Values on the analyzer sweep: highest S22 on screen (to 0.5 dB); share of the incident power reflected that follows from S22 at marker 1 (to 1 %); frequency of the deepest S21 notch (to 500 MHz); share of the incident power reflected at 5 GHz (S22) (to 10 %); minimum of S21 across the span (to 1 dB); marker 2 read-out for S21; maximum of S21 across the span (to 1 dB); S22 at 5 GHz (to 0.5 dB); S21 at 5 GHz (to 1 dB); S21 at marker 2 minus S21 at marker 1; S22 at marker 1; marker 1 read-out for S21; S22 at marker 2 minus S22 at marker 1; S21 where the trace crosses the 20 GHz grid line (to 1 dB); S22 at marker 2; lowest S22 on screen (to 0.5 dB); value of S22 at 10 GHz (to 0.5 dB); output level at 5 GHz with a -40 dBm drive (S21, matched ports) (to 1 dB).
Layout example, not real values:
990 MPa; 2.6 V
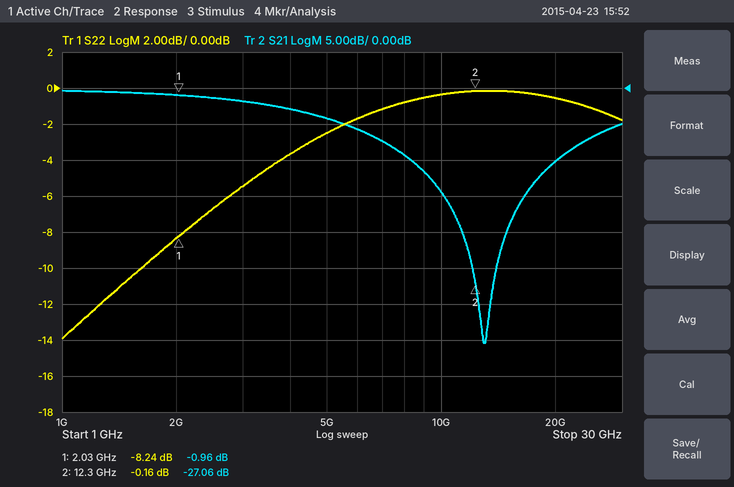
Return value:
0.0 dB; 15 %; 13.0 GHz; 60 %; -35 dB; -27.06 dB; 0 dB; -2.5 dB; -4 dB; -26.10 dB; -8.24 dB; -0.96 dB; 8.08 dB; -10 dB; -0.16 dB; -14.0 dB; -0.5 dB; -44 dBm
